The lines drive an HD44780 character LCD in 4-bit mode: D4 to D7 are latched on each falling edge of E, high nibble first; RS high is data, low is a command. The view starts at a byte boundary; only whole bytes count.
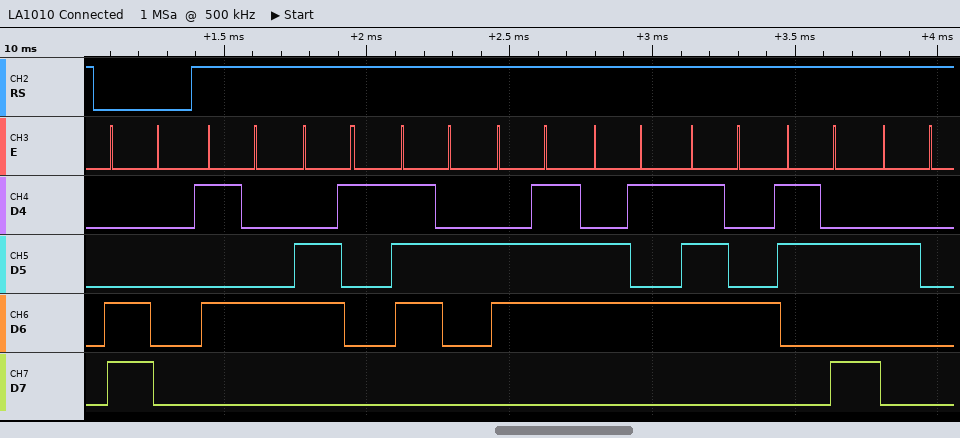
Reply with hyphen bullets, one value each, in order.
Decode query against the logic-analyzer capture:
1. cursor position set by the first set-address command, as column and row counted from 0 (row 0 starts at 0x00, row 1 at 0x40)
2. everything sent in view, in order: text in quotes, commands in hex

- column 0, row 1
- 0xC0 "Target: "
